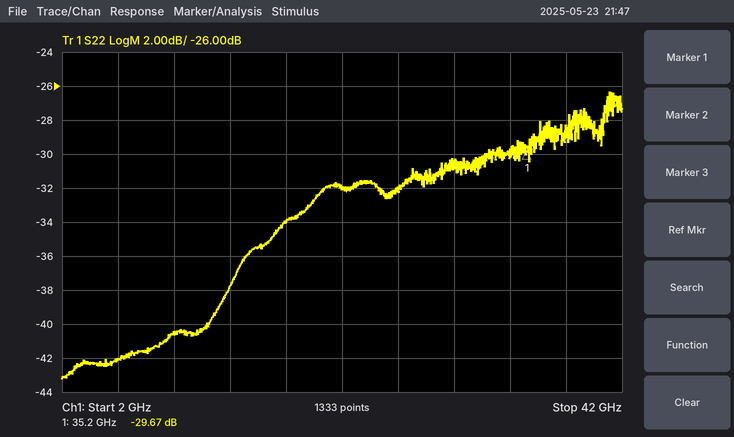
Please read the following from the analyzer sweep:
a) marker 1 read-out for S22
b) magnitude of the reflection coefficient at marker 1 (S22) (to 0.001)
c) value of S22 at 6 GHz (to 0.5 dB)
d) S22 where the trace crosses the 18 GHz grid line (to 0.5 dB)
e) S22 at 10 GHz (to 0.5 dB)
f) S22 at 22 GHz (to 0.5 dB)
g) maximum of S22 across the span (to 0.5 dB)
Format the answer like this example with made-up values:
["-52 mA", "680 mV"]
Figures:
["-29.67 dB", "0.033", "-42.0 dB", "-34.0 dB", "-40.5 dB", "-32.0 dB", "-26.5 dB"]
